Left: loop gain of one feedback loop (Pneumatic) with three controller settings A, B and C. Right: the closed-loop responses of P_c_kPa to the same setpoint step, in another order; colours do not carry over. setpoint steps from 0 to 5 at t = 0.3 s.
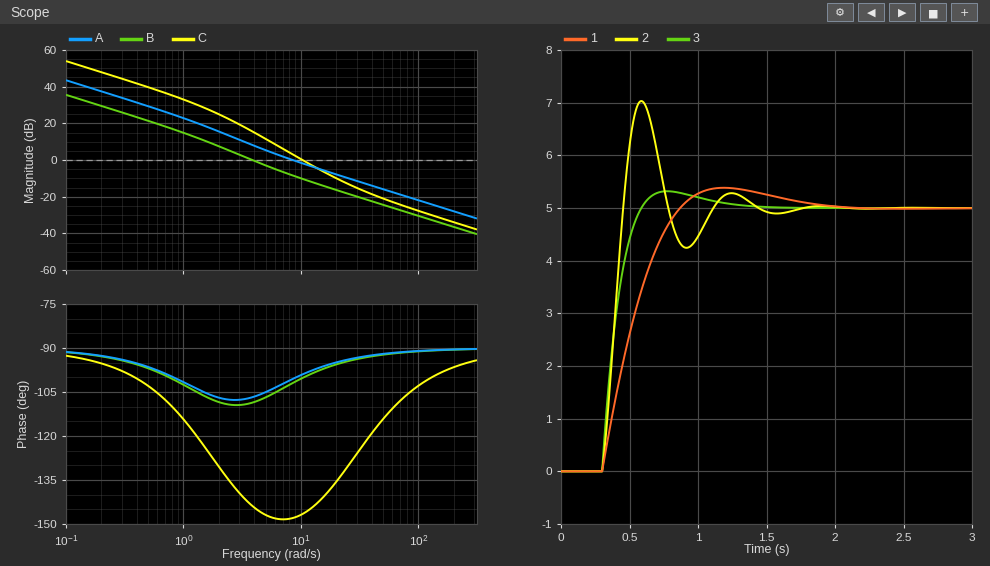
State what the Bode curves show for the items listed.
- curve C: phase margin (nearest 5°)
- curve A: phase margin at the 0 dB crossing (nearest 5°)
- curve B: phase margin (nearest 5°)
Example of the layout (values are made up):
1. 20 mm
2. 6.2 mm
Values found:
1. 35°
2. 80°
3. 70°
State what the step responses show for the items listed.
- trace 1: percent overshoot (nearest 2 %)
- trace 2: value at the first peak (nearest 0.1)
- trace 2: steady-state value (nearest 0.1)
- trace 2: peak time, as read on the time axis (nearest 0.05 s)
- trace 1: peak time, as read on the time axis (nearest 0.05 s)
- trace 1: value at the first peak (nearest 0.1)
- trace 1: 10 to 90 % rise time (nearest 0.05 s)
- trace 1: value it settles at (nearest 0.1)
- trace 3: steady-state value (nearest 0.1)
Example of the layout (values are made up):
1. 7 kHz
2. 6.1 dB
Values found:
1. 8 %
2. 7.0
3. 5.0
4. 0.60 s
5. 1.20 s
6. 5.4
7. 0.40 s
8. 5.0
9. 5.0
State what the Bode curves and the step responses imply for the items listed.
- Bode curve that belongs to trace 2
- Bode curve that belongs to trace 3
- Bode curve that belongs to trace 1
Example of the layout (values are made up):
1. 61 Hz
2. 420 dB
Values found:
1. C
2. A
3. B
